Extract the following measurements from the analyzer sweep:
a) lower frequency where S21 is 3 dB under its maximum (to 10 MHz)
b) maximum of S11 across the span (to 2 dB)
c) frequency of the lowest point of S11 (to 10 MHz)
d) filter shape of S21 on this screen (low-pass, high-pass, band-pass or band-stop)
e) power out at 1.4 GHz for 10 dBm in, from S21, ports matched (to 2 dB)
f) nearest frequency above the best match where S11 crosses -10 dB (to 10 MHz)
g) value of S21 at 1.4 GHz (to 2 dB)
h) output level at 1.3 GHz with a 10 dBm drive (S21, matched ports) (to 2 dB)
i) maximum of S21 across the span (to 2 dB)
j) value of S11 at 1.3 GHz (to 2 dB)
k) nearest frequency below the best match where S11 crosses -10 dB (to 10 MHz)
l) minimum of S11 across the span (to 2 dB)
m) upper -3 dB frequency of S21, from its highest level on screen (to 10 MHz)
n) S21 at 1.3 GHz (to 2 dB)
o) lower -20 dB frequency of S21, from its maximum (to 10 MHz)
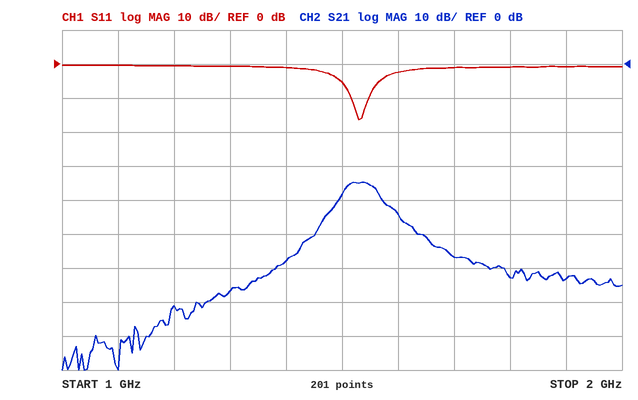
1.50 GHz
0 dB
1.53 GHz
band-pass
-48 dBm
1.55 GHz
-58 dB
-56 dBm
-34 dB
0 dB
1.52 GHz
-16 dB
1.56 GHz
-66 dB
1.42 GHz
